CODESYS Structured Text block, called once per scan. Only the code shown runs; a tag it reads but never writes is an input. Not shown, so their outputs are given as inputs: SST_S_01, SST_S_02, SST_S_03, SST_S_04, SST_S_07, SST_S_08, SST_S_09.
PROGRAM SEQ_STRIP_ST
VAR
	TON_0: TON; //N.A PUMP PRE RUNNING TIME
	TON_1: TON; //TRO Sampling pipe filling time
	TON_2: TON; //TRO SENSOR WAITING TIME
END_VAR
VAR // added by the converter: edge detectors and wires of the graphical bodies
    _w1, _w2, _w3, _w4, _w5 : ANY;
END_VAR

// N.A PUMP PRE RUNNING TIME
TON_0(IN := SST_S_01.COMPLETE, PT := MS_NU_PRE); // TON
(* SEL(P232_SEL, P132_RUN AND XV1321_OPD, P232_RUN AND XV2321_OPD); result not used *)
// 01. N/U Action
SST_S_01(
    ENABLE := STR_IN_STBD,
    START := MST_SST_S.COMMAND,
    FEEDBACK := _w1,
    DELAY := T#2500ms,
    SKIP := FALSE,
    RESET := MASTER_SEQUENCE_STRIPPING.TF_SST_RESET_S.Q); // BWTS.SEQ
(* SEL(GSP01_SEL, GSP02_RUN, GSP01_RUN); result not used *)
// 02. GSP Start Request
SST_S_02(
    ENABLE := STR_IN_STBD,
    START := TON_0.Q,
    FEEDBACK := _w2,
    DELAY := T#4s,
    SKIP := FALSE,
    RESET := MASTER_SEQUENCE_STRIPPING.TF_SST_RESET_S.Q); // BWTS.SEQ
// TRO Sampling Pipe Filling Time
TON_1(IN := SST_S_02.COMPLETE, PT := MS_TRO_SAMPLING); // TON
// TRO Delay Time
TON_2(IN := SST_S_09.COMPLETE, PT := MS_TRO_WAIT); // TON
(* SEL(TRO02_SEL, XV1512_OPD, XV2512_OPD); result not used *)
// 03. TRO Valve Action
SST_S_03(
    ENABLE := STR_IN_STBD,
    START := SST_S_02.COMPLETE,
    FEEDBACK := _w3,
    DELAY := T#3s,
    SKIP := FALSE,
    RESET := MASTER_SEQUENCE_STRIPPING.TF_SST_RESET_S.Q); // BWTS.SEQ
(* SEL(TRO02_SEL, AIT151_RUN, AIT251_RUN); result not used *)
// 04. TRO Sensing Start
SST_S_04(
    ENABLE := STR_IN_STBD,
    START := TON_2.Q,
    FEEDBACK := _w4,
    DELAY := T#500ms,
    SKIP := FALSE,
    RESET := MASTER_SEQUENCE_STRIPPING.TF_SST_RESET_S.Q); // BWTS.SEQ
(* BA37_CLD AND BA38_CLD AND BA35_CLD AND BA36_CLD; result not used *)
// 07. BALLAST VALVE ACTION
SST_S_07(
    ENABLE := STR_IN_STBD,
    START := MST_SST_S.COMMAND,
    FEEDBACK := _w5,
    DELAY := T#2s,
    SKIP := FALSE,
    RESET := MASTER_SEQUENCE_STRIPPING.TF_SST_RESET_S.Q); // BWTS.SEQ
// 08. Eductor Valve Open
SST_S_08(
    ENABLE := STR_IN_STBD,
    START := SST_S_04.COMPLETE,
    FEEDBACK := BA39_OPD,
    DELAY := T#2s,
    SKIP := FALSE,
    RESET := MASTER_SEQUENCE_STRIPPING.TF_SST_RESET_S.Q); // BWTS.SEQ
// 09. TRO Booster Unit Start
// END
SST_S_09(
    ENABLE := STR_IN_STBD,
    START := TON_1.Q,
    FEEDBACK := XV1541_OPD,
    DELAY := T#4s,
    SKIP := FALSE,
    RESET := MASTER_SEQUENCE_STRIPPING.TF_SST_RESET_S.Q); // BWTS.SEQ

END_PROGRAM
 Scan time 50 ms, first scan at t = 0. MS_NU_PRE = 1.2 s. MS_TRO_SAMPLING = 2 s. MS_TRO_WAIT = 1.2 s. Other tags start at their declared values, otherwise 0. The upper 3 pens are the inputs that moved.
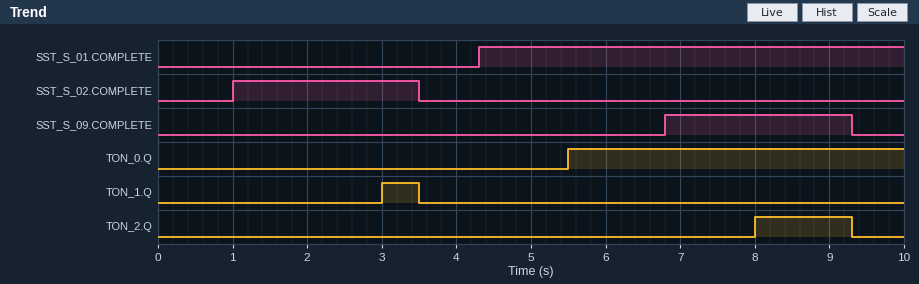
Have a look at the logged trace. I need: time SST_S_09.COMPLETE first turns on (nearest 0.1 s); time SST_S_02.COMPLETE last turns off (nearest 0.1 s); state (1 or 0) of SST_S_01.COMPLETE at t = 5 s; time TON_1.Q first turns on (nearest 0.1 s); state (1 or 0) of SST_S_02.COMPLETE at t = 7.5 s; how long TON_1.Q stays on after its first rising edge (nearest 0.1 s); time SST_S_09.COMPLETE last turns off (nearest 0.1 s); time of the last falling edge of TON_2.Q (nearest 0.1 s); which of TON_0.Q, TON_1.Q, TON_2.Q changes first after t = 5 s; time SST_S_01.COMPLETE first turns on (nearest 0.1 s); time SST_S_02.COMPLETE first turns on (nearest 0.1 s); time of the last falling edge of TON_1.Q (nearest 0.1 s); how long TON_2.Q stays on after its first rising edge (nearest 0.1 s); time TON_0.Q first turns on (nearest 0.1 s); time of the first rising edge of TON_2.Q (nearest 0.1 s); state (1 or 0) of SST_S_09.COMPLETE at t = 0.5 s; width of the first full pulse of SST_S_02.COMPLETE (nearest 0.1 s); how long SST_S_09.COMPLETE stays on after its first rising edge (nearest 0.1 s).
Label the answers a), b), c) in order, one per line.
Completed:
a) 6.8 s
b) 3.5 s
c) 1
d) 3.0 s
e) 0
f) 0.5 s
g) 9.3 s
h) 9.3 s
i) TON_0.Q
j) 4.3 s
k) 1.0 s
l) 3.5 s
m) 1.3 s
n) 5.5 s
o) 8.0 s
p) 0
q) 2.5 s
r) 2.5 s
